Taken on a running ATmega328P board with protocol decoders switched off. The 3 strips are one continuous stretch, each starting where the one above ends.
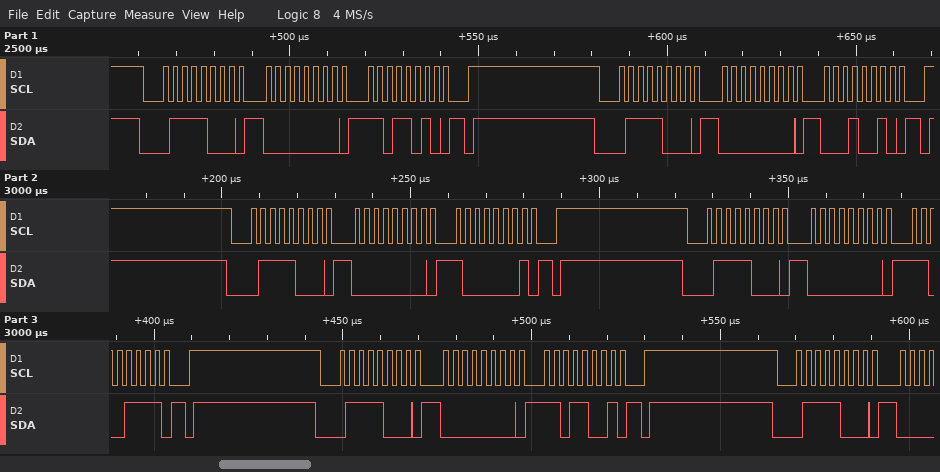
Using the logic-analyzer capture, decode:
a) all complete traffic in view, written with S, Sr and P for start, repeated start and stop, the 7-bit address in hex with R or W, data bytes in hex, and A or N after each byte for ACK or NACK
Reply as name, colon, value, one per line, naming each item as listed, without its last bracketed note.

all complete traffic in view, written with S, Sr and P for start, repeated start and stop, the 7-bit address in hex with R or W, data bytes in hex, and A or N after each byte for ACK or NACK: S 3CW A 00 A DA A P S 3CW A 00 A 12 A P S 3CW A 00 A 81 A P S 3CW A 00 A CF A P S 3CW A 00 A D9 A P S 3CW A
